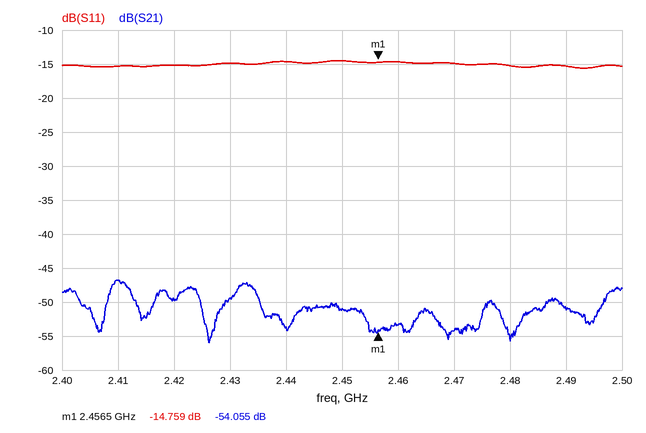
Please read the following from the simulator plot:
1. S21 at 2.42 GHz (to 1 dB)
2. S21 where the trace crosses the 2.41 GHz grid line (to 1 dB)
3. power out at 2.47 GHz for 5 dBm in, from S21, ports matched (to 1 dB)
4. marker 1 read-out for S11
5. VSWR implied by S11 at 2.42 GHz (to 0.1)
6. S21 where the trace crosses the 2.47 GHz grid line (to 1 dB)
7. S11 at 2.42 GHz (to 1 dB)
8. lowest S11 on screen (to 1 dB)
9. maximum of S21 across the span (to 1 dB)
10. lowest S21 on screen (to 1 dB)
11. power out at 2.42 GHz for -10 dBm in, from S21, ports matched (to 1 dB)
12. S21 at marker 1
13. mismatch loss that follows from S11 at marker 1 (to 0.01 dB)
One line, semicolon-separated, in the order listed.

-50 dB; -47 dB; -49 dBm; -14.759 dB; 1.4; -54 dB; -15 dB; -16 dB; -47 dB; -56 dB; -60 dBm; -54.055 dB; 0.15 dB
